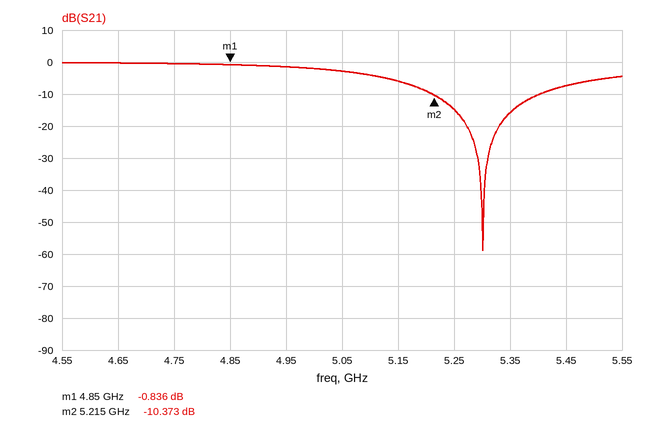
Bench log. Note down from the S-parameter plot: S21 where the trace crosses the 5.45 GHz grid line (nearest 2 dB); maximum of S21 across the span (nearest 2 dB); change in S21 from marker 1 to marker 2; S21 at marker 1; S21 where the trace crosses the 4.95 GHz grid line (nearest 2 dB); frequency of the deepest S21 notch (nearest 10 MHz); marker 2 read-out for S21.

-8 dB
0 dB
-9.537 dB
-0.836 dB
-2 dB
5.30 GHz
-10.373 dB
